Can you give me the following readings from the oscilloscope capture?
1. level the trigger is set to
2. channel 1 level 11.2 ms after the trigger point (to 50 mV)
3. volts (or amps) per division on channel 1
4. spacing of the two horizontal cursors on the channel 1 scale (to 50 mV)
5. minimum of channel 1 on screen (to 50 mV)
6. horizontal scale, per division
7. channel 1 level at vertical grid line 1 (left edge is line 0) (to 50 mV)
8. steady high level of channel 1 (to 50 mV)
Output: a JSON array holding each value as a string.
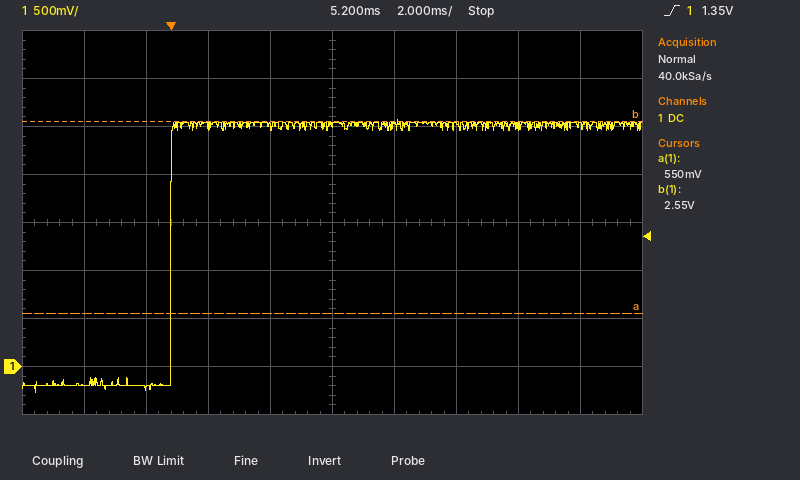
["1.35 V", "2.50 V", "500 mV", "2.00 V", "-250 mV", "2 ms", "-200 mV", "2.55 V"]
